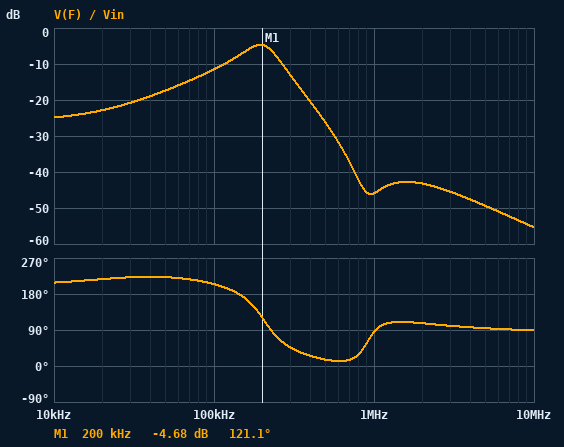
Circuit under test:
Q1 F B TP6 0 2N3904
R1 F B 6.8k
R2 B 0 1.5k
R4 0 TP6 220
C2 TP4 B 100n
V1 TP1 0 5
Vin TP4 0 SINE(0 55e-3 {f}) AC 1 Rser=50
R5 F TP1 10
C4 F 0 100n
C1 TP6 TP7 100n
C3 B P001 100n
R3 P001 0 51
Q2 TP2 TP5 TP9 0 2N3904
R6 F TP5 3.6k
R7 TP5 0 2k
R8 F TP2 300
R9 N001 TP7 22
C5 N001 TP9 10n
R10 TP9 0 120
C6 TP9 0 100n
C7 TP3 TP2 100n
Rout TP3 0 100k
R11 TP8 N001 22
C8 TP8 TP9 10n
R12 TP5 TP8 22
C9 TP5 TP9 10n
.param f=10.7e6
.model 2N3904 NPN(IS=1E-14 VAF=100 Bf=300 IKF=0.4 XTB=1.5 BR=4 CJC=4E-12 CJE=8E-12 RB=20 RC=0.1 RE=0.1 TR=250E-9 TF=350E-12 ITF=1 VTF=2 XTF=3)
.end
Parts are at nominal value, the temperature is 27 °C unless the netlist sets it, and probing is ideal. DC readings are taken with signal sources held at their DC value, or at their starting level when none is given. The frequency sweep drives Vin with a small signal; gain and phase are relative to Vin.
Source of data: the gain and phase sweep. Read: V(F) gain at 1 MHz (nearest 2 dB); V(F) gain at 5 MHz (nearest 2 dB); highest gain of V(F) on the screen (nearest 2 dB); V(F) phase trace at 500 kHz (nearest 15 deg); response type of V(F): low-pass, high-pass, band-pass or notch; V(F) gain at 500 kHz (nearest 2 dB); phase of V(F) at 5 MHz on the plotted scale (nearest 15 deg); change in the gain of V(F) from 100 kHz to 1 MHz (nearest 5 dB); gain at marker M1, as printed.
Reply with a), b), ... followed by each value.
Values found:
a) -46 dB
b) -50 dB
c) -4 dB
d) 15 deg
e) band-pass
f) -26 dB
g) 90 deg
h) -35 dB
i) -4.68 dB
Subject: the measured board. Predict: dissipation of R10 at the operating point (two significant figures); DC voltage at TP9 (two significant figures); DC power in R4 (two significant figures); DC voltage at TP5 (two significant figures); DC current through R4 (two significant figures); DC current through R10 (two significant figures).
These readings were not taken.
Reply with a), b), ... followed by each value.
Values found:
a) 8.3 mW
b) 1.0 V
c) 230 µW
d) 1.7 V
e) 1.0 mA
f) 8.3 mA
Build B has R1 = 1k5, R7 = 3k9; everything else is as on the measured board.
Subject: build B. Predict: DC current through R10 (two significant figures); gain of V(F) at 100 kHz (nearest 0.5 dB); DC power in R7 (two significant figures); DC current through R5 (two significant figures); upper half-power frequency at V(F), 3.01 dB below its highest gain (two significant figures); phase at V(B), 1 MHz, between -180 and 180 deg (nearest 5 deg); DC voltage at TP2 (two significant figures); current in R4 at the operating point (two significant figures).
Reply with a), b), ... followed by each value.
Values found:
a) 11 mA
b) -25.0 dB
c) 1.1 mW
d) 21 mA
e) 380 kHz
f) 0 deg
g) 1.4 V
h) 7.6 mA
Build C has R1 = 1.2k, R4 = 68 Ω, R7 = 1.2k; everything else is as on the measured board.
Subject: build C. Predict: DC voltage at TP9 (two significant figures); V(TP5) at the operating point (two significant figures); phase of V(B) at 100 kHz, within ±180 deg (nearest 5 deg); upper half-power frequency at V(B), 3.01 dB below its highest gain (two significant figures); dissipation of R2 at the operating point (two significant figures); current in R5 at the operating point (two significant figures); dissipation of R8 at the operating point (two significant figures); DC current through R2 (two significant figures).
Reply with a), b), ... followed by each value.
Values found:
a) 470 mV
b) 1.2 V
c) 0 deg
d) 210 MHz
e) 4.3 mW
f) 33 mA
g) 4.5 mW
h) 1.7 mA
